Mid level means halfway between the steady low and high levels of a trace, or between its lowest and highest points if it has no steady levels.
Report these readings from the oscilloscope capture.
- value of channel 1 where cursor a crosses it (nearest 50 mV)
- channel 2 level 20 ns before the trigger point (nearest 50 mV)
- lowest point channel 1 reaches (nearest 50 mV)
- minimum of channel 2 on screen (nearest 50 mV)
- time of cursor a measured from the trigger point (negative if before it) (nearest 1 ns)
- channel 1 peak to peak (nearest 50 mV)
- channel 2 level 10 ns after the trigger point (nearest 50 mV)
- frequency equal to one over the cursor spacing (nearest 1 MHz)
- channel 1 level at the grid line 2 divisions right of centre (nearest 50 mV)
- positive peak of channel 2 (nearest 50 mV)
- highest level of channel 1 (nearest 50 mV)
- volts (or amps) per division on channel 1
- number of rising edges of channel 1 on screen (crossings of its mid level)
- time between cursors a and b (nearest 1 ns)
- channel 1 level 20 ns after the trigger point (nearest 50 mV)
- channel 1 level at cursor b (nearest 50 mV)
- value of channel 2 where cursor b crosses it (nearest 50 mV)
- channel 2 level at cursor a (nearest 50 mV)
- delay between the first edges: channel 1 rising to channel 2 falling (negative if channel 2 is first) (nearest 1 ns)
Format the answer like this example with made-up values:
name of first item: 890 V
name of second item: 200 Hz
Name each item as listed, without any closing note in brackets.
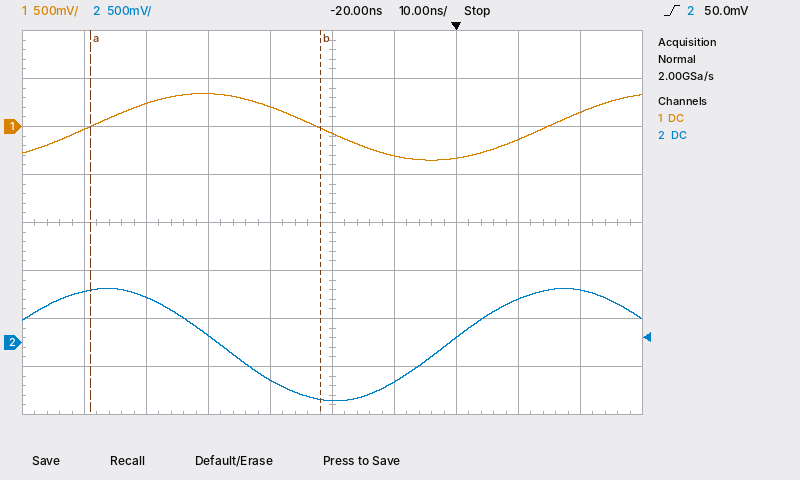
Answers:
value of channel 1 where cursor a crosses it: 0 mV
channel 2 level 20 ns before the trigger point: -600 mV
lowest point channel 1 reaches: -350 mV
minimum of channel 2 on screen: -600 mV
time of cursor a measured from the trigger point (negative if before it): -59 ns
channel 1 peak to peak: 700 mV
channel 2 level 10 ns after the trigger point: 450 mV
frequency equal to one over the cursor spacing: 27 MHz
channel 1 level at the grid line 2 divisions right of centre: -350 mV
positive peak of channel 2: 550 mV
highest level of channel 1: 350 mV
volts (or amps) per division on channel 1: 500 mV
number of rising edges of channel 1 on screen: 2
time between cursors a and b: 37 ns
channel 1 level 20 ns after the trigger point: 150 mV
channel 1 level at cursor b: 0 mV
value of channel 2 where cursor b crosses it: -600 mV
channel 2 level at cursor a: 550 mV
delay between the first edges: channel 1 rising to channel 2 falling (negative if channel 2 is first): +21 ns
